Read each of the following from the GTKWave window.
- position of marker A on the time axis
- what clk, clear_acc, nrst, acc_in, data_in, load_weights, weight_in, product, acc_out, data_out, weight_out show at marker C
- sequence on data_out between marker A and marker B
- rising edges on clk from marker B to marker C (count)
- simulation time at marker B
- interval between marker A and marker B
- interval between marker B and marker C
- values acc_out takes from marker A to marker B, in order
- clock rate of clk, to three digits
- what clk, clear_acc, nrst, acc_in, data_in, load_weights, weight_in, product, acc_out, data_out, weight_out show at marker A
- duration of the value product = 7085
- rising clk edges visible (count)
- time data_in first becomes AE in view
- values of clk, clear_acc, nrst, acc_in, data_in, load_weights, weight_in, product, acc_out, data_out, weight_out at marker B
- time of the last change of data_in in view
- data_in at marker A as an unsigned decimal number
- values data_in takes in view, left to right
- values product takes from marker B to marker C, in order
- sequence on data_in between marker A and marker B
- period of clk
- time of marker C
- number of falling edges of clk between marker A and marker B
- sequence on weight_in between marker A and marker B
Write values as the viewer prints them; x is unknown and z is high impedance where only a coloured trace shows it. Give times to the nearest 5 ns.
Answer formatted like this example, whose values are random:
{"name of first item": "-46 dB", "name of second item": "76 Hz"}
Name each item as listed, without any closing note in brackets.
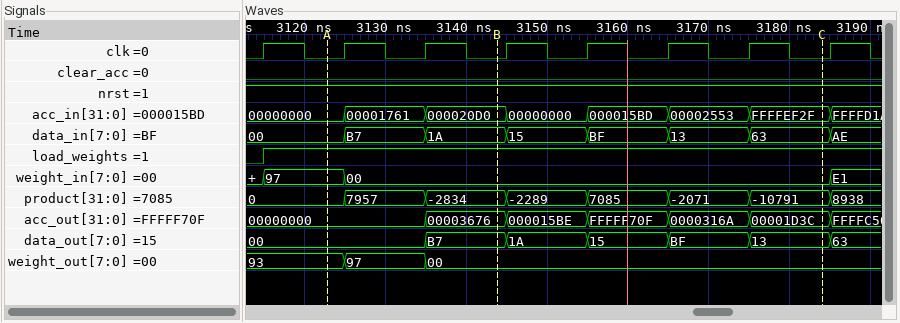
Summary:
{"position of marker A on the time axis": "3125 ns", "what clk, clear_acc, nrst, acc_in, data_in, load_weights, weight_in, product, acc_out, data_out, weight_out show at marker C": "clk=0, clear_acc=0, nrst=1, acc_in=FFFFEF2F, data_in=63, load_weights=1, weight_in=00, product=-10791, acc_out=00001D3C, data_out=13, weight_out=00", "sequence on data_out between marker A and marker B": "00, B7", "rising edges on clk from marker B to marker C": "4", "simulation time at marker B": "3145 ns", "interval between marker A and marker B": "20 ns", "interval between marker B and marker C": "40 ns", "values acc_out takes from marker A to marker B, in order": "00000000, 00003676", "clock rate of clk, to three digits": "100 MHz", "what clk, clear_acc, nrst, acc_in, data_in, load_weights, weight_in, product, acc_out, data_out, weight_out show at marker A": "clk=0, clear_acc=0, nrst=1, acc_in=00000000, data_in=00, load_weights=1, weight_in=97, product=0, acc_out=00000000, data_out=00, weight_out=93", "duration of the value product = 7085": "10 ns", "rising clk edges visible": "8", "time data_in first becomes AE in view": "3185 ns", "values of clk, clear_acc, nrst, acc_in, data_in, load_weights, weight_in, product, acc_out, data_out, weight_out at marker B": "clk=0, clear_acc=0, nrst=1, acc_in=000020D0, data_in=1A, load_weights=1, weight_in=00, product=-2834, acc_out=00003676, data_out=B7, weight_out=00", "time of the last change of data_in in view": "3185 ns", "data_in at marker A as an unsigned decimal number": "0", "values data_in takes in view, left to right": "00, B7, 1A, 15, BF, 13, 63, AE", "values product takes from marker B to marker C, in order": "-2834, -2289, 7085, -2071, -10791", "sequence on data_in between marker A and marker B": "00, B7, 1A", "period of clk": "10 ns", "time of marker C": "3185 ns", "number of falling edges of clk between marker A and marker B": "2", "sequence on weight_in between marker A and marker B": "97, 00"}
